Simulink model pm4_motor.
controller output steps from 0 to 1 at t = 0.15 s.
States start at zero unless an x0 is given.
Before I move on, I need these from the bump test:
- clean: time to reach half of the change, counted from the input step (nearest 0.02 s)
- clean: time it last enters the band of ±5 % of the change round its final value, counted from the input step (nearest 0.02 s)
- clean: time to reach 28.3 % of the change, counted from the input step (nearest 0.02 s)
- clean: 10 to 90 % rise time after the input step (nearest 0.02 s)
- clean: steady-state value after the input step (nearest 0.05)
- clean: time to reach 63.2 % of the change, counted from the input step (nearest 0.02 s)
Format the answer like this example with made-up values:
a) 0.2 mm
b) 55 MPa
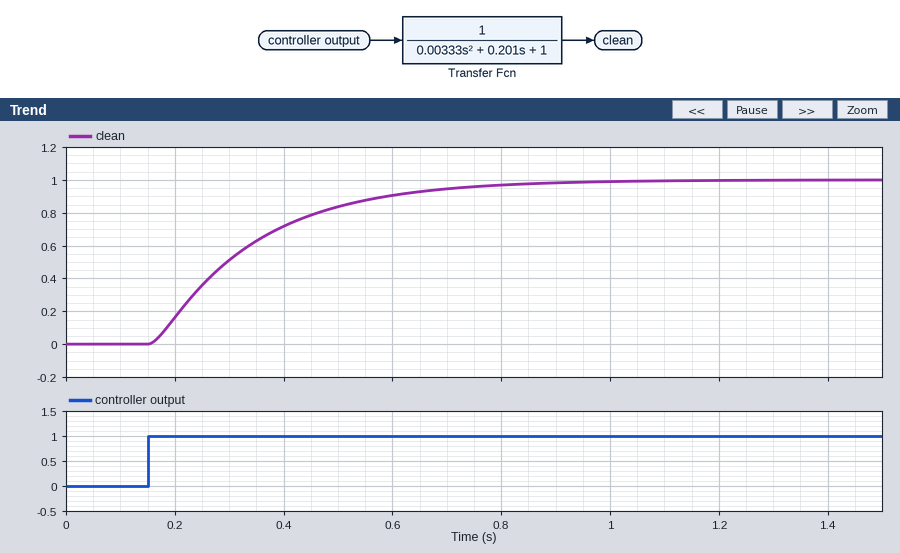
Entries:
a) 0.14 s
b) 0.56 s
c) 0.08 s
d) 0.40 s
e) 1.00
f) 0.20 s
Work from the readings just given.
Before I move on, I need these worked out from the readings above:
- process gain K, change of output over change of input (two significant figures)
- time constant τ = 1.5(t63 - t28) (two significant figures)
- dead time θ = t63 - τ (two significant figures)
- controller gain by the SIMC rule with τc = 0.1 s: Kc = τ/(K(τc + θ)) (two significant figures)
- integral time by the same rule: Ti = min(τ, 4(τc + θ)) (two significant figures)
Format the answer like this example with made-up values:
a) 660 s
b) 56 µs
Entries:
a) 1.0
b) 0.18 s
c) 0.020 s
d) 1.5
e) 0.18 s
